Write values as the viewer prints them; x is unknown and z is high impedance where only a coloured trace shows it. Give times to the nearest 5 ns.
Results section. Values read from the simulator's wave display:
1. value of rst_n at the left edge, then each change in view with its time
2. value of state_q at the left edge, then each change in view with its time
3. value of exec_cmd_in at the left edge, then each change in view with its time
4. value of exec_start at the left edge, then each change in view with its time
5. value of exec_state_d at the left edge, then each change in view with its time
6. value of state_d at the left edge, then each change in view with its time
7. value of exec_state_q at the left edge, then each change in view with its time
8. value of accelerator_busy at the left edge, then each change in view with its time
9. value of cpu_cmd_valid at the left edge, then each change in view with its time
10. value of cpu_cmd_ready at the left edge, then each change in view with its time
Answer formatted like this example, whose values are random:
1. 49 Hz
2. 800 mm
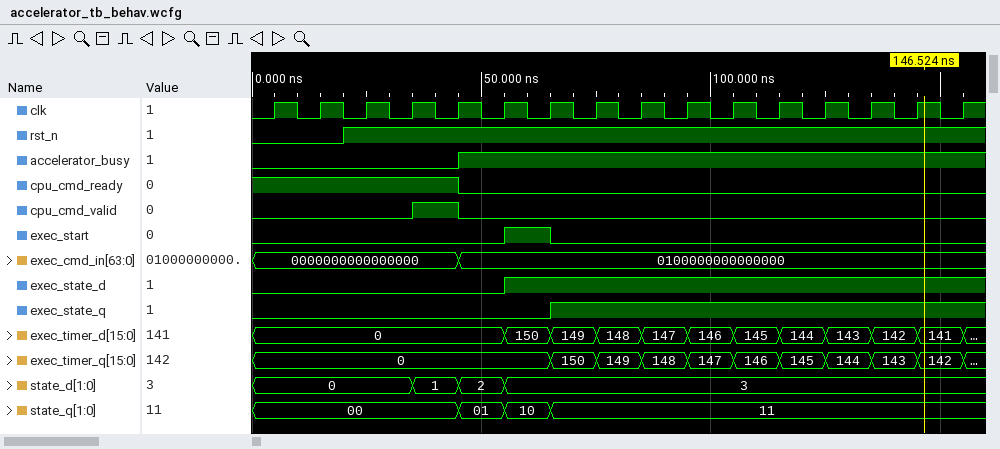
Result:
1. 0, 1 at 20 ns
2. 00, 01 at 45 ns, 10 at 55 ns, 11 at 65 ns
3. 0000000000000000, 0100000000000000 at 45 ns
4. 0, 1 at 55 ns, 0 at 65 ns
5. 0, 1 at 55 ns
6. 0, 1 at 35 ns, 2 at 45 ns, 3 at 55 ns
7. 0, 1 at 65 ns
8. 0, 1 at 45 ns
9. 0, 1 at 35 ns, 0 at 45 ns
10. 1, 0 at 45 ns
